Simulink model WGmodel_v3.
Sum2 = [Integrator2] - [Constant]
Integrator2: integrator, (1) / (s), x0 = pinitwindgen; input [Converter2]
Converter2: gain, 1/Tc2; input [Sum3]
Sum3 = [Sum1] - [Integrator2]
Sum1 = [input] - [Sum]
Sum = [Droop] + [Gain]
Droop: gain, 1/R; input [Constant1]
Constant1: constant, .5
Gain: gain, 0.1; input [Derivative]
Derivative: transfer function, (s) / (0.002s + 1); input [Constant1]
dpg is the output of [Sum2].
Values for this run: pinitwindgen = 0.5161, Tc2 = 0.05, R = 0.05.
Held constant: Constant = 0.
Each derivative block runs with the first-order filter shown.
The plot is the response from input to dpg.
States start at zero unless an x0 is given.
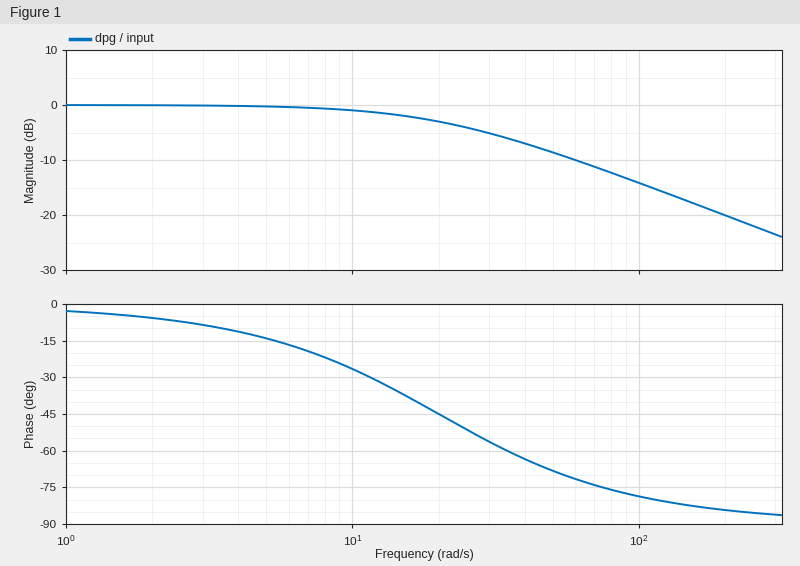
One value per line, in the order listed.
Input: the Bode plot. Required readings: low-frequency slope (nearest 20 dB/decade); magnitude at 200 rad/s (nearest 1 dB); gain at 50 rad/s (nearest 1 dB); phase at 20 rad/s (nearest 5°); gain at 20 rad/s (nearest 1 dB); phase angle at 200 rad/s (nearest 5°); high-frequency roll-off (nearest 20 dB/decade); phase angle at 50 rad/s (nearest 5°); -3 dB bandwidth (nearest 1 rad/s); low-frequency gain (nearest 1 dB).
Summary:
0 dB/decade
-20 dB
-9 dB
-45°
-3 dB
-85°
-20 dB/decade
-70°
20 rad/s
0 dB
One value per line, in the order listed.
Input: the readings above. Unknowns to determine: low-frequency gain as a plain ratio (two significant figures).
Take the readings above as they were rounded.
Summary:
1.0
